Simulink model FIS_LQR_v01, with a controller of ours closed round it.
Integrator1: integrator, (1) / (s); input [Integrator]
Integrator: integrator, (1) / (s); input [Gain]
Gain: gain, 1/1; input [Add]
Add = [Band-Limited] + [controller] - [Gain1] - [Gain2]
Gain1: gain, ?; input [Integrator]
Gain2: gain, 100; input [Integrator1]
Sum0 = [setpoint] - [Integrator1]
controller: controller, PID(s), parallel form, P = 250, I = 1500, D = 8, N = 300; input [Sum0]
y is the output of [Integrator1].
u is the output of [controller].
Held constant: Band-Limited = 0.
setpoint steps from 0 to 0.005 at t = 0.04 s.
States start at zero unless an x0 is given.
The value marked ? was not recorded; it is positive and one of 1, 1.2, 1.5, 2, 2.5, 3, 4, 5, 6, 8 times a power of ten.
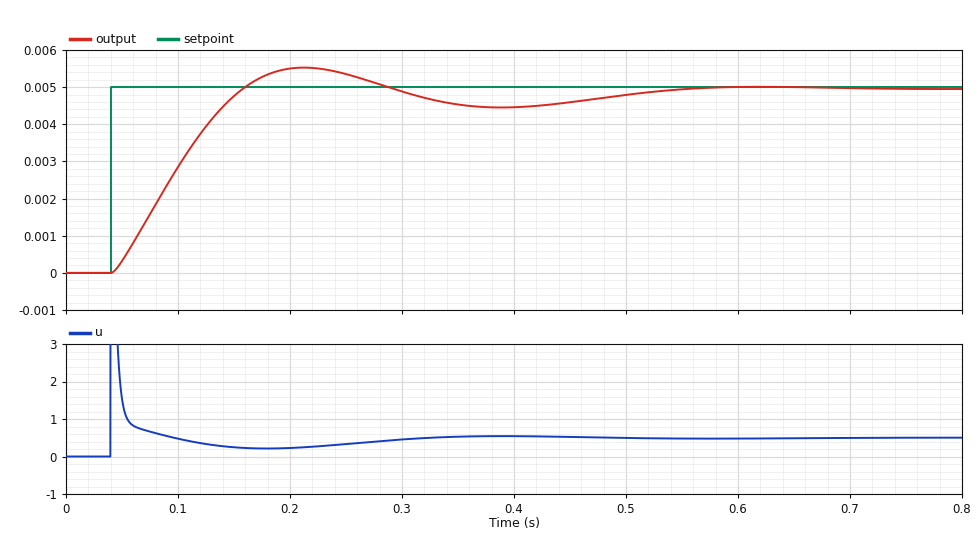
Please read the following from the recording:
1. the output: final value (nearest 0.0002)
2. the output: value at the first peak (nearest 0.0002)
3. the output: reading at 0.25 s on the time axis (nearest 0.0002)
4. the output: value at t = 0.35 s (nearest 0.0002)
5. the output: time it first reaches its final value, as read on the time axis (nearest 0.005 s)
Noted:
0.0050
0.0056
0.0054
0.0046
0.160 s
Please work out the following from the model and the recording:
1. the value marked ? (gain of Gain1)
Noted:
10
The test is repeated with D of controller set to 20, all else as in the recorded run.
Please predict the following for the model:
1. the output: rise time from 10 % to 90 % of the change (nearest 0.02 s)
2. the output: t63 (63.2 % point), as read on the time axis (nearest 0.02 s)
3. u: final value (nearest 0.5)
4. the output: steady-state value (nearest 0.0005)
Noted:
0.10 s
0.08 s
0.5
0.0050
